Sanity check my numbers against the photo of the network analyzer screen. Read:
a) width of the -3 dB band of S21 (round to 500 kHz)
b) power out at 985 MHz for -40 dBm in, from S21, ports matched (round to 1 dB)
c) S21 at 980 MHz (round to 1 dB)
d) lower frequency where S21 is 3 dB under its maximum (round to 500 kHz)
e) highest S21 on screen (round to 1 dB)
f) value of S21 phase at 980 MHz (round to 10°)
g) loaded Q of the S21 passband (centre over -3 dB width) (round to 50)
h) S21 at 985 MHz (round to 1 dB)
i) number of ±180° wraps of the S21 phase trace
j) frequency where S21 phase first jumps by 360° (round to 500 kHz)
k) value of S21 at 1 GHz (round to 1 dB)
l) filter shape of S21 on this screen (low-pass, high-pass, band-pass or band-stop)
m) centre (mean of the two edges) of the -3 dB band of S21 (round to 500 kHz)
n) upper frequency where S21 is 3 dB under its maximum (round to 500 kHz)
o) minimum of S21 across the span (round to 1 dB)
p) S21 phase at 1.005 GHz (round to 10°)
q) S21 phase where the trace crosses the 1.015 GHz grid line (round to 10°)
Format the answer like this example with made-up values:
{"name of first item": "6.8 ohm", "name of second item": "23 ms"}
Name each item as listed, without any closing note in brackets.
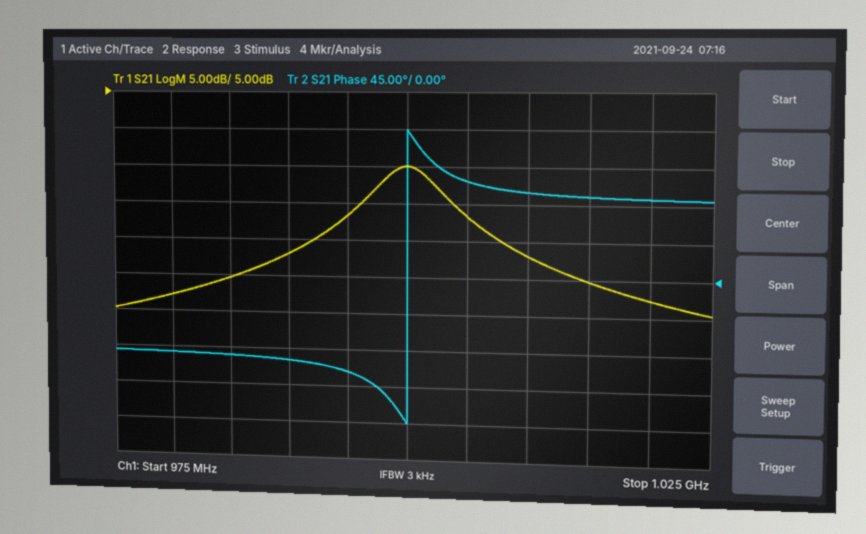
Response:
{"width of the -3 dB band of S21": "5.0 MHz", "power out at 985 MHz for -40 dBm in, from S21, ports matched": "-60 dBm", "S21 at 980 MHz": "-23 dB", "lower frequency where S21 is 3 dB under its maximum": "997.5 MHz", "highest S21 on screen": "-5 dB", "value of S21 phase at 980 MHz": "-100°", "loaded Q of the S21 passband (centre over -3 dB width)": "200", "S21 at 985 MHz": "-20 dB", "number of ±180° wraps of the S21 phase trace": "1", "frequency where S21 phase first jumps by 360°": "1.0000 GHz", "value of S21 at 1 GHz": "-5 dB", "filter shape of S21 on this screen": "band-pass", "centre (mean of the two edges) of the -3 dB band of S21": "1.0000 GHz", "upper frequency where S21 is 3 dB under its maximum": "1.0025 GHz", "minimum of S21 across the span": "-25 dB", "S21 phase at 1.005 GHz": "120°", "S21 phase where the trace crosses the 1.015 GHz grid line": "100°"}
